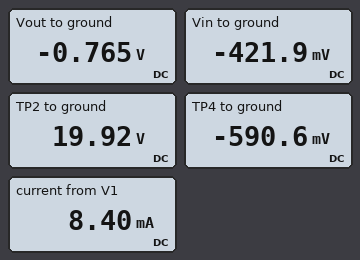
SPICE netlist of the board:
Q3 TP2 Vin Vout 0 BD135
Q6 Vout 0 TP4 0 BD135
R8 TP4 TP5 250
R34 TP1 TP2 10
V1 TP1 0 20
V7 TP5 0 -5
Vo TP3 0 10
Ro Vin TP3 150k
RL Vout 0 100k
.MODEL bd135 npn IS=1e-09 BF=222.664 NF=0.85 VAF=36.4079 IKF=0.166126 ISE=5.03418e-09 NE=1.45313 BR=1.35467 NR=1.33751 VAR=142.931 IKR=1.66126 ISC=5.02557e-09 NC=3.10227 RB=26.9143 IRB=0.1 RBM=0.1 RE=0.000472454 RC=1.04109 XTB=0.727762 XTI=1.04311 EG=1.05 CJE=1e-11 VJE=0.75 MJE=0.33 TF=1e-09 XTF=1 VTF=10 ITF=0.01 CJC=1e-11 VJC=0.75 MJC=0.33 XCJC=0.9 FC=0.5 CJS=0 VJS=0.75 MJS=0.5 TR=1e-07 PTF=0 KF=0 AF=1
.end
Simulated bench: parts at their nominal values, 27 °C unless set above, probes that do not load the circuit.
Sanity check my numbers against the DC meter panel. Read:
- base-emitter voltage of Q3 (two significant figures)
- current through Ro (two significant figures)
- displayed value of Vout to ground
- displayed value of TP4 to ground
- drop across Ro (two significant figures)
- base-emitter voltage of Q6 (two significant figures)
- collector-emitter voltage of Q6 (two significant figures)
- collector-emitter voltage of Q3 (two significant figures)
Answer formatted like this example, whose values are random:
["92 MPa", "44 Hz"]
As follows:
["340 mV", "69 µA", "-0.765 V", "-590.6 mV", "10 V", "590 mV", "-170 mV", "21 V"]
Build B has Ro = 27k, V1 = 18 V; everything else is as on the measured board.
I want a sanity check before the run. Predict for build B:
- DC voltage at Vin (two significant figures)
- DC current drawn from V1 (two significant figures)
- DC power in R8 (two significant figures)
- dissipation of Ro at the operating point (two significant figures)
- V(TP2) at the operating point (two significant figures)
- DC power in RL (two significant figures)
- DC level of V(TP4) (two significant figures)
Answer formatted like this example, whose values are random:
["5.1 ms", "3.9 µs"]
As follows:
["6.0 V", "18 mA", "86 mW", "580 µW", "18 V", "320 µW", "-370 mV"]
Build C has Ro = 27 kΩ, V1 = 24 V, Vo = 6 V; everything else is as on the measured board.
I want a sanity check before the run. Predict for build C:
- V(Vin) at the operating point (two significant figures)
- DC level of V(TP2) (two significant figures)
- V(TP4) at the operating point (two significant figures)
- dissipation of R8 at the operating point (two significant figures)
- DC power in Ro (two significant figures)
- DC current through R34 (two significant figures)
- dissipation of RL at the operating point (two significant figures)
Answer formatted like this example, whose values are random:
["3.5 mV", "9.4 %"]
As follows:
["2.6 V", "24 V", "-370 mV", "86 mW", "430 µW", "18 mA", "50 µW"]
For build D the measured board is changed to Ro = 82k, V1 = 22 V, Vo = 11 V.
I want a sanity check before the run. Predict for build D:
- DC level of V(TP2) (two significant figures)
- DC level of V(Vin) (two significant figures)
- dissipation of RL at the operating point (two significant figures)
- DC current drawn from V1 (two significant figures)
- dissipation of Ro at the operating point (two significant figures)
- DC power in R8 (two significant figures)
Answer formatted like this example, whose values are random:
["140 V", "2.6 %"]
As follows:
["22 V", "660 mV", "890 nW", "18 mA", "1.3 mW", "86 mW"]
